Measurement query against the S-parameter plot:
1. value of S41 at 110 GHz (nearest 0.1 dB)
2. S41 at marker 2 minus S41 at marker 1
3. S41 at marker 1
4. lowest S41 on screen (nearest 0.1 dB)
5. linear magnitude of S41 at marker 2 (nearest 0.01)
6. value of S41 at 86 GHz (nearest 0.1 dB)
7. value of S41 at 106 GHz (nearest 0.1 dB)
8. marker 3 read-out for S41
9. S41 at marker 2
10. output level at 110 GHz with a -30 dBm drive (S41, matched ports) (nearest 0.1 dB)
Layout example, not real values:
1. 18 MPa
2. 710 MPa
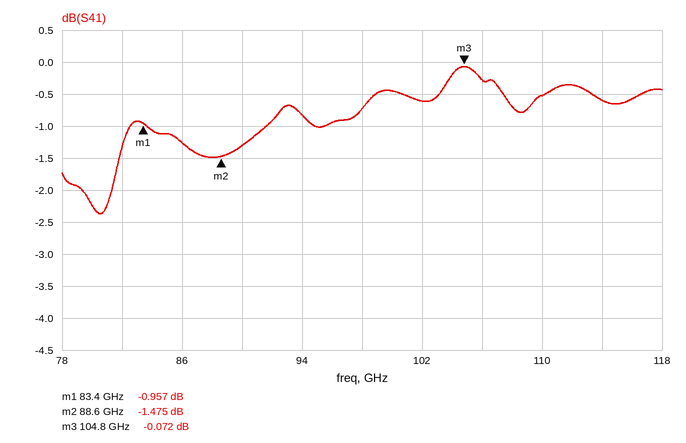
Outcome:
1. -0.5 dB
2. -0.518 dB
3. -0.957 dB
4. -2.4 dB
5. 0.84
6. -1.3 dB
7. -0.3 dB
8. -0.072 dB
9. -1.475 dB
10. -30.5 dBm
